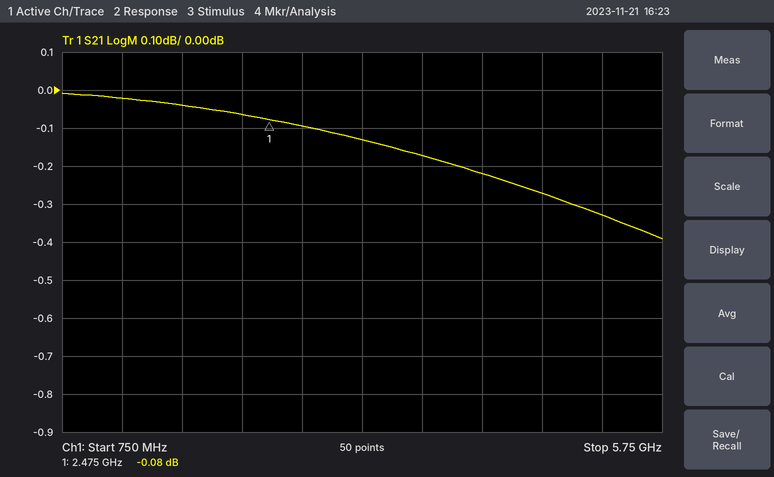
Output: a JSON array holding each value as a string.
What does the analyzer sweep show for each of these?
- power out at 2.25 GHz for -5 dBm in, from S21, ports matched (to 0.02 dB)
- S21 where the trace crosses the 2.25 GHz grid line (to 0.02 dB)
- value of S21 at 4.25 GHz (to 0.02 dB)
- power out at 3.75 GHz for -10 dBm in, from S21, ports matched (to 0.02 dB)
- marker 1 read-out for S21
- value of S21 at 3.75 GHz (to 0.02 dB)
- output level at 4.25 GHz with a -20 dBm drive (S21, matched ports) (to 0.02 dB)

["-5.06 dBm", "-0.06 dB", "-0.22 dB", "-10.18 dBm", "-0.08 dB", "-0.18 dB", "-20.22 dBm"]
